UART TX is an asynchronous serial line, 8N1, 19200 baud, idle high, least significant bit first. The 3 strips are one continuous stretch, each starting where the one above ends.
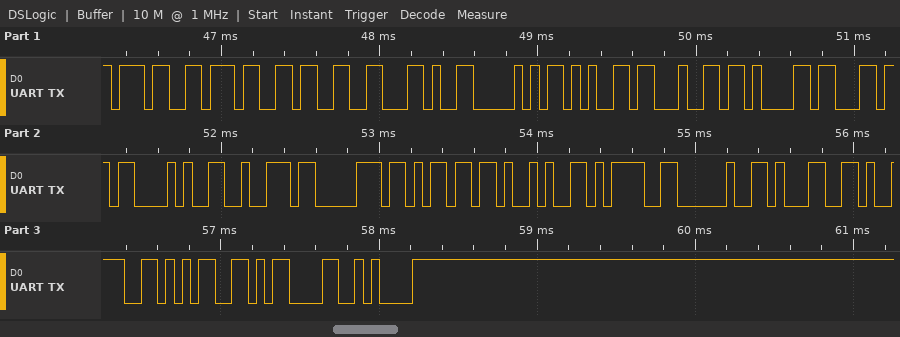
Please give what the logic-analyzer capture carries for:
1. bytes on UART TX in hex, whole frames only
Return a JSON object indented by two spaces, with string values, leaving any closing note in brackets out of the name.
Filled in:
{
  "bytes on UART TX in hex, whole frames only": "0x37 0x37 0x33 0x2C 0x50 0x65 0x64 0x61 0x6C 0x28 0x72 0x70 0x6D 0x29 0x3D 0x20 0x31 0x39 0x35 0x0D 0x0A"
}
